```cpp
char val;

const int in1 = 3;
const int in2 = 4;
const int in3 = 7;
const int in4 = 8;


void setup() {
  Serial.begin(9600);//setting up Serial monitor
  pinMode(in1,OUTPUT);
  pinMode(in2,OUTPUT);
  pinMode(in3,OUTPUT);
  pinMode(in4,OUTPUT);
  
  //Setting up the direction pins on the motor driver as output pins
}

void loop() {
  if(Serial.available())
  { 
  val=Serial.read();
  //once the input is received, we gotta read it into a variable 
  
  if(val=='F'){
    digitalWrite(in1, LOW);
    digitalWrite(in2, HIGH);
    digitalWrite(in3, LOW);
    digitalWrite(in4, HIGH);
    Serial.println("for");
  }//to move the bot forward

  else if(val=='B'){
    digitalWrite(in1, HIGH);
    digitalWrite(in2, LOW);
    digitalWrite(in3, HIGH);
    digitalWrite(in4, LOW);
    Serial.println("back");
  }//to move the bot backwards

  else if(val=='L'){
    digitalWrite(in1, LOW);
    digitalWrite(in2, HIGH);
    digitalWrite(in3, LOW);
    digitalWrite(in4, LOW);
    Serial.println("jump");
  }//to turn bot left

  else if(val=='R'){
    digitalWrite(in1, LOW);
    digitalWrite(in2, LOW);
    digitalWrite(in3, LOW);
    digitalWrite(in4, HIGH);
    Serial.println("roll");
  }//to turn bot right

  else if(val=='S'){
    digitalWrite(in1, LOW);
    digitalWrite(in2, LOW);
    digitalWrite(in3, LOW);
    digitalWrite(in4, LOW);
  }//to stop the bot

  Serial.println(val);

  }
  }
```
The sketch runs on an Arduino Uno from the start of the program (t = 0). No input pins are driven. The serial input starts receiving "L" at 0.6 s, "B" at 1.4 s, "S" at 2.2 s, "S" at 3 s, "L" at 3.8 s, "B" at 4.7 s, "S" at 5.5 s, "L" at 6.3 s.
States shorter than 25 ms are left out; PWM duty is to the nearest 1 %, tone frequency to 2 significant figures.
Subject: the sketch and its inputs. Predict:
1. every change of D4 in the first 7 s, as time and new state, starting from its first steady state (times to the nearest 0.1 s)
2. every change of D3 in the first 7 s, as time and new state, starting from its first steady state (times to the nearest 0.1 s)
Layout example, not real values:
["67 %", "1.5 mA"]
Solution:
["0 s low; 0.6 s high; 1.4 s low; 3.8 s high; 4.7 s low; 6.3 s high", "0 s low; 1.4 s high; 2.2 s low; 4.7 s high; 5.5 s low"]
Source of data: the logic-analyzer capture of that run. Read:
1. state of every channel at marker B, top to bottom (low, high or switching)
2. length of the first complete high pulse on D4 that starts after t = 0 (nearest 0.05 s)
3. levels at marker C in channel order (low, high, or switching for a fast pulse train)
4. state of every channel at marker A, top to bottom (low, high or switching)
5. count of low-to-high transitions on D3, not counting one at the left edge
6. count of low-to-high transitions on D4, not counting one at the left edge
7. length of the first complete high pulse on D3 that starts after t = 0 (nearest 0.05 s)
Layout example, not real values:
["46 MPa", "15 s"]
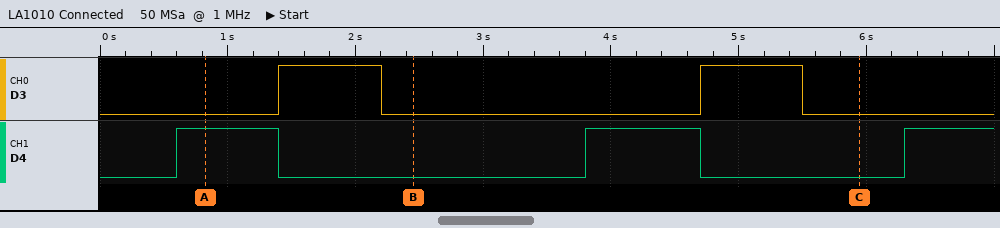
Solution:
["D3 low, D4 low", "0.80 s", "D3 low, D4 low", "D3 low, D4 high", "2", "3", "0.80 s"]
